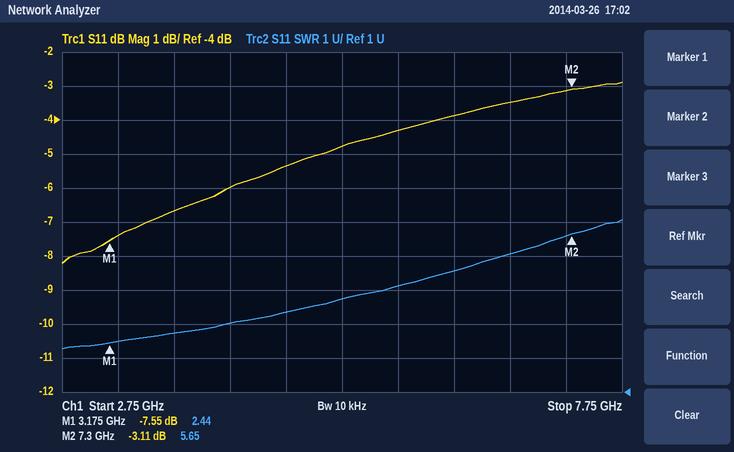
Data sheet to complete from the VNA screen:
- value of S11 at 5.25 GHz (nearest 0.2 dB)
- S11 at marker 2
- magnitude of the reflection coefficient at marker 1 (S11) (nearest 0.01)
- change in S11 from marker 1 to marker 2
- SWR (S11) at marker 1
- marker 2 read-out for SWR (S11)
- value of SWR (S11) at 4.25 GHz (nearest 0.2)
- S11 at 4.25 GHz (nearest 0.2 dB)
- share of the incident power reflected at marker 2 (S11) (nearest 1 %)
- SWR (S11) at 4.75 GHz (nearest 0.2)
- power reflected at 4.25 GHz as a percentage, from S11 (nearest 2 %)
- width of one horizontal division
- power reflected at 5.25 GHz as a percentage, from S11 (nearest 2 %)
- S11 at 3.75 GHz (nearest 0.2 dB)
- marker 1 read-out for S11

-4.8 dB
-3.11 dB
0.42
4.44 dB
2.44
5.65
3.0
-6.0 dB
49 %
3.4
26 %
500 MHz
34 %
-6.6 dB
-7.55 dB
